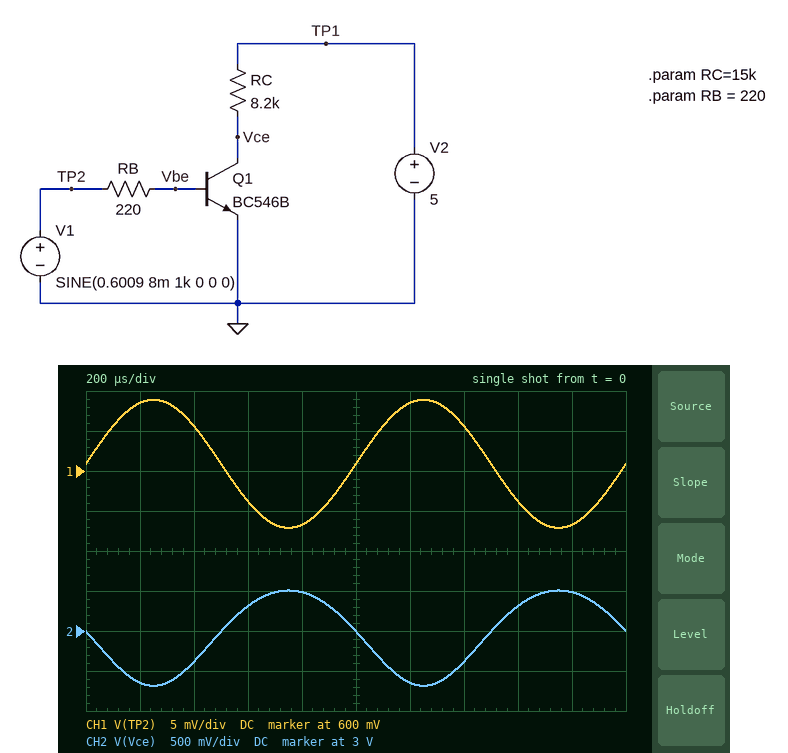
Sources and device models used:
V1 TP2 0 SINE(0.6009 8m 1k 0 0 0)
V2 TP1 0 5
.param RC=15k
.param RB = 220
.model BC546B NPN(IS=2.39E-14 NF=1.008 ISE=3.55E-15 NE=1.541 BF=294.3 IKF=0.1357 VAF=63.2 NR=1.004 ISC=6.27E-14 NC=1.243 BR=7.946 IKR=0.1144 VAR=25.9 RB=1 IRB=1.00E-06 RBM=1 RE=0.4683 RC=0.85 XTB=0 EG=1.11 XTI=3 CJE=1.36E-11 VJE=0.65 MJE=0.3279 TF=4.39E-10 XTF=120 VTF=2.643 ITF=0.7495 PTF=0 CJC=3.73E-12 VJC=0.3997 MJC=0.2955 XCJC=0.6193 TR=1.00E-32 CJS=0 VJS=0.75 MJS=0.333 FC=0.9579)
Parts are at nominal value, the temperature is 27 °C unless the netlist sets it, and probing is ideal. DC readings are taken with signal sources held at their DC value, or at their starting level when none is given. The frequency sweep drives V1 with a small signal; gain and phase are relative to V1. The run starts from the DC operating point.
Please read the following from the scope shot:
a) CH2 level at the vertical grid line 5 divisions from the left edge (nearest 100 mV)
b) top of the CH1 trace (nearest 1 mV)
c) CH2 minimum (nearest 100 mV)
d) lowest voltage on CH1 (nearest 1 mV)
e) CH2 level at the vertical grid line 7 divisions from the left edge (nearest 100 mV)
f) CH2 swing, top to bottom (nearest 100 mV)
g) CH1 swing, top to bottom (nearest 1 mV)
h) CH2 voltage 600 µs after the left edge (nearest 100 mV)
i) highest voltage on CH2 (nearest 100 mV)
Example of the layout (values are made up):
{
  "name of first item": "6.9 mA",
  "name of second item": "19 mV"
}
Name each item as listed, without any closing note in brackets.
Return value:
{
  "CH2 level at the vertical grid line 5 divisions from the left edge": "3.0 V",
  "top of the CH1 trace": "609 mV",
  "CH2 minimum": "2.3 V",
  "lowest voltage on CH1": "593 mV",
  "CH2 level at the vertical grid line 7 divisions from the left edge": "2.6 V",
  "CH2 swing, top to bottom": "1.2 V",
  "CH1 swing, top to bottom": "16 mV",
  "CH2 voltage 600 µs after the left edge": "3.3 V",
  "highest voltage on CH2": "3.5 V"
}
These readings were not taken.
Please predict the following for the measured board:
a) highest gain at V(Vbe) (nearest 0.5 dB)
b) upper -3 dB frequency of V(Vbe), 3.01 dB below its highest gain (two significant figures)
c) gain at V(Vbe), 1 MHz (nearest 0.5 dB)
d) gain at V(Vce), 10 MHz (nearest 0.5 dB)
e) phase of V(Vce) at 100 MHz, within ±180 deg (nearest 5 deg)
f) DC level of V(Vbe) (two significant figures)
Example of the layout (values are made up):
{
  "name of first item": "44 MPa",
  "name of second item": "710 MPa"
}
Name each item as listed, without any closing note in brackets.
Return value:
{
  "highest gain at V(Vbe)": "0 dB",
  "upper -3 dB frequency of V(Vbe), 3.01 dB below its highest gain": "3.1 MHz",
  "gain at V(Vbe), 1 MHz": "-0.5 dB",
  "gain at V(Vce), 10 MHz": "26.0 dB",
  "phase of V(Vce) at 100 MHz, within ±180 deg": "30 deg",
  "DC level of V(Vbe)": "600 mV"
}
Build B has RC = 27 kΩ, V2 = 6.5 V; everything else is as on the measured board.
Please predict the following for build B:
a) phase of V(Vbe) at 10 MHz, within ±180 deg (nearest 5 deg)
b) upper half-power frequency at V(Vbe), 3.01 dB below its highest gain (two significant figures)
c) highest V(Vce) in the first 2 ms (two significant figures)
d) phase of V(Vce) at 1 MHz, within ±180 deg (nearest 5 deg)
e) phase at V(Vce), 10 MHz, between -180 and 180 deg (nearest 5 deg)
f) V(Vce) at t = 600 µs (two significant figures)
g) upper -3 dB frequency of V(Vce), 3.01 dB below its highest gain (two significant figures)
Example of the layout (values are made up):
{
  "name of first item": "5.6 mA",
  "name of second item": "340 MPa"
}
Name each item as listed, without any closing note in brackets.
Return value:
{
  "phase of V(Vbe) at 10 MHz, within ±180 deg": "-10 deg",
  "upper half-power frequency at V(Vbe), 3.01 dB below its highest gain": "230 kHz",
  "highest V(Vce) in the first 2 ms": "1.7 V",
  "phase of V(Vce) at 1 MHz, within ±180 deg": "100 deg",
  "phase at V(Vce), 10 MHz, between -180 and 180 deg": "75 deg",
  "V(Vce) at t = 600 µs": "1.1 V",
  "upper -3 dB frequency of V(Vce), 3.01 dB below its highest gain": "200 kHz"
}
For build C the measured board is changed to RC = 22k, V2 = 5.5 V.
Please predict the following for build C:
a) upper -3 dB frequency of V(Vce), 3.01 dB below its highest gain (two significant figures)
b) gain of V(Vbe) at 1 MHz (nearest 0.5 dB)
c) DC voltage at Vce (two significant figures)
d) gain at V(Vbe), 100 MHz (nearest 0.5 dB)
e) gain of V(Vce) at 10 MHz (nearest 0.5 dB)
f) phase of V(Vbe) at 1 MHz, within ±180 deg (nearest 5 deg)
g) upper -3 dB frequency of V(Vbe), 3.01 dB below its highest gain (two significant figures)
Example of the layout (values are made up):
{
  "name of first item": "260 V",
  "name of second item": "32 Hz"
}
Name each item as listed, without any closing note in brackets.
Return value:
{
  "upper -3 dB frequency of V(Vce), 3.01 dB below its highest gain": "510 kHz",
  "gain of V(Vbe) at 1 MHz": "-5.5 dB",
  "DC voltage at Vce": "340 mV",
  "gain at V(Vbe), 100 MHz": "-15.0 dB",
  "gain of V(Vce) at 10 MHz": "19.0 dB",
  "phase of V(Vbe) at 1 MHz, within ±180 deg": "-30 deg",
  "upper -3 dB frequency of V(Vbe), 3.01 dB below its highest gain": "580 kHz"
}
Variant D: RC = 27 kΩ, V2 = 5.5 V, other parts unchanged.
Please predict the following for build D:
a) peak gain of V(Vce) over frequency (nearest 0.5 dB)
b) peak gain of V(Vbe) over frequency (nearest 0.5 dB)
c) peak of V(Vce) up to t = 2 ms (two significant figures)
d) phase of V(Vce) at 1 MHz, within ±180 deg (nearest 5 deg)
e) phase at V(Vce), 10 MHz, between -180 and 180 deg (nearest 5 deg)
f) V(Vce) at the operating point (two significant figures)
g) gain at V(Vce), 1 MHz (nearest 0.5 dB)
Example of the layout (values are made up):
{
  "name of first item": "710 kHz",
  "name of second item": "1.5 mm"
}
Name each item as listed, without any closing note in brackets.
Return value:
{
  "peak gain of V(Vce) over frequency": "15.5 dB",
  "peak gain of V(Vbe) over frequency": "-2.0 dB",
  "peak of V(Vce) up to t = 2 ms": "790 mV",
  "phase of V(Vce) at 1 MHz, within ±180 deg": "150 deg",
  "phase at V(Vce), 10 MHz, between -180 and 180 deg": "75 deg",
  "V(Vce) at the operating point": "64 mV",
  "gain at V(Vce), 1 MHz": "14.5 dB"
}
